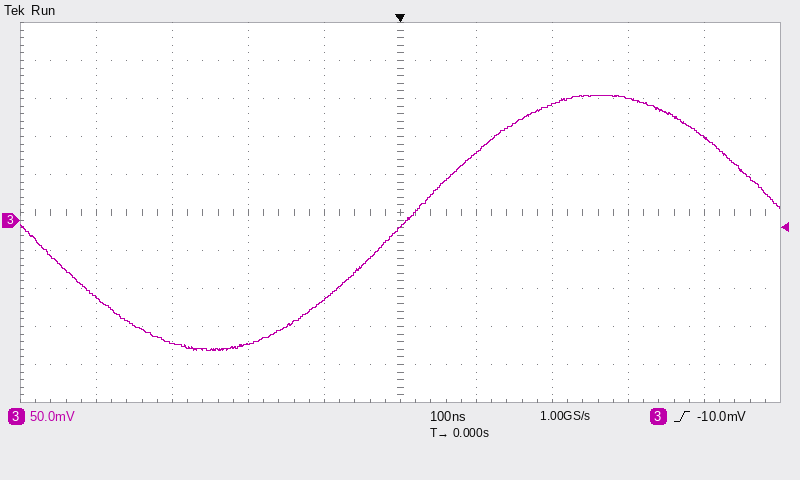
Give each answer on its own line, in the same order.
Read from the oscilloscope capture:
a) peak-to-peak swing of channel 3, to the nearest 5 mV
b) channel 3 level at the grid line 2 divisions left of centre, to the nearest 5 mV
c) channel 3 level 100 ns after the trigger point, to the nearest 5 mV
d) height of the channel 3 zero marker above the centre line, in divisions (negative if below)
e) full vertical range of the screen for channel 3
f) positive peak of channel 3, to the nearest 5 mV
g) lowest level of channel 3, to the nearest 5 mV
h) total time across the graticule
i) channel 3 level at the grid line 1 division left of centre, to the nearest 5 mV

335 mV
-165 mV
90 mV
-0.2 div
500 mV
165 mV
-170 mV
1 µs
-105 mV
